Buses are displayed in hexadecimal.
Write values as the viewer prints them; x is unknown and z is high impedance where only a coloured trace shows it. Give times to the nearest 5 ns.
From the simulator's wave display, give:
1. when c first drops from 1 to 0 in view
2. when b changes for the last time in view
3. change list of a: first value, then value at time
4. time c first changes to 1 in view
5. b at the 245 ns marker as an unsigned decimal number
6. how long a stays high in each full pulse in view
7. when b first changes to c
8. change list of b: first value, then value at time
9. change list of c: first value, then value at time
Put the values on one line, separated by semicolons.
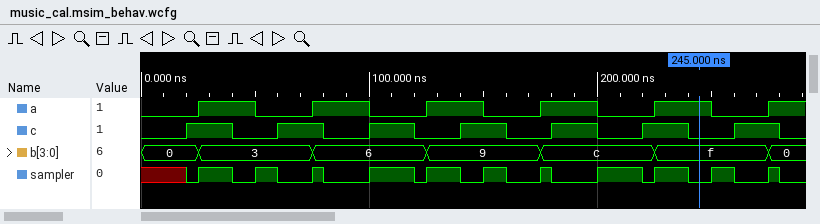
40 ns; 275 ns; 0, 1 at 25 ns, 0 at 50 ns, 1 at 75 ns, 0 at 100 ns, 1 at 125 ns, 0 at 150 ns, 1 at 175 ns, 0 at 200 ns, 1 at 225 ns, 0 at 250 ns, 1 at 275 ns; 20 ns; 15; 25 ns, 25 ns, 25 ns, 25 ns, 25 ns; 175 ns; 0, 3 at 25 ns, 6 at 75 ns, 9 at 125 ns, c at 175 ns, f at 225 ns, 0 at 275 ns; 0, 1 at 20 ns, 0 at 40 ns, 1 at 60 ns, 0 at 80 ns, 1 at 100 ns, 0 at 120 ns, 1 at 140 ns, 0 at 160 ns, 1 at 180 ns, 0 at 200 ns, 1 at 220 ns, 0 at 240 ns, 1 at 260 ns, 0 at 280 ns
